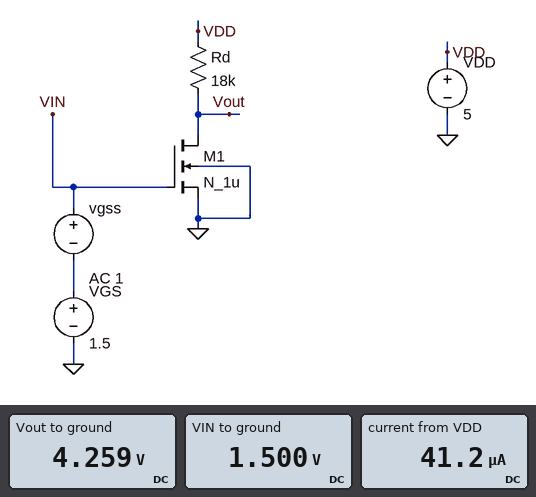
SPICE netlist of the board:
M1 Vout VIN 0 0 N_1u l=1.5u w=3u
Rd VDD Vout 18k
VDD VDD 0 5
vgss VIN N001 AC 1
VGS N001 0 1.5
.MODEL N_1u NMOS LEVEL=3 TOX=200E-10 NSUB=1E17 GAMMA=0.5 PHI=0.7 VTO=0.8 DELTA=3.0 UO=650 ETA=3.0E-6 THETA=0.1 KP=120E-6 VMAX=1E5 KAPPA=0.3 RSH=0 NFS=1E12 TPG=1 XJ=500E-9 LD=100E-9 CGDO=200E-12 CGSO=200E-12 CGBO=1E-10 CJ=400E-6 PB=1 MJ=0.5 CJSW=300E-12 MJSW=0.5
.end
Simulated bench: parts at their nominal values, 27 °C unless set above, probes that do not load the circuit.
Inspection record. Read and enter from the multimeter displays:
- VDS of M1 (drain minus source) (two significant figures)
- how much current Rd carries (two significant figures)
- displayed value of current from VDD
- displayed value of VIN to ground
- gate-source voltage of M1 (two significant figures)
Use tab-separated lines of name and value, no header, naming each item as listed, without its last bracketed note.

VDS of M1 (drain minus source)	4.3 V
how much current Rd carries	41 µA
displayed value of current from VDD	41.2 µA
displayed value of VIN to ground	1.500 V
gate-source voltage of M1	1.5 V
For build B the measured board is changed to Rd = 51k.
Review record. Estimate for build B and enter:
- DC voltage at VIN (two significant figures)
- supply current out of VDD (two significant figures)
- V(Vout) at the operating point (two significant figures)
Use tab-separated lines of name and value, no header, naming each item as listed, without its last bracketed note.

DC voltage at VIN	1.5 V
supply current out of VDD	40 µA
V(Vout) at the operating point	2.9 V
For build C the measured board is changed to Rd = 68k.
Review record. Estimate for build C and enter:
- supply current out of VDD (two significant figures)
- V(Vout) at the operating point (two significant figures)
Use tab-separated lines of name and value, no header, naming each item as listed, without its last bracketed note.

supply current out of VDD	40 µA
V(Vout) at the operating point	2.3 V
